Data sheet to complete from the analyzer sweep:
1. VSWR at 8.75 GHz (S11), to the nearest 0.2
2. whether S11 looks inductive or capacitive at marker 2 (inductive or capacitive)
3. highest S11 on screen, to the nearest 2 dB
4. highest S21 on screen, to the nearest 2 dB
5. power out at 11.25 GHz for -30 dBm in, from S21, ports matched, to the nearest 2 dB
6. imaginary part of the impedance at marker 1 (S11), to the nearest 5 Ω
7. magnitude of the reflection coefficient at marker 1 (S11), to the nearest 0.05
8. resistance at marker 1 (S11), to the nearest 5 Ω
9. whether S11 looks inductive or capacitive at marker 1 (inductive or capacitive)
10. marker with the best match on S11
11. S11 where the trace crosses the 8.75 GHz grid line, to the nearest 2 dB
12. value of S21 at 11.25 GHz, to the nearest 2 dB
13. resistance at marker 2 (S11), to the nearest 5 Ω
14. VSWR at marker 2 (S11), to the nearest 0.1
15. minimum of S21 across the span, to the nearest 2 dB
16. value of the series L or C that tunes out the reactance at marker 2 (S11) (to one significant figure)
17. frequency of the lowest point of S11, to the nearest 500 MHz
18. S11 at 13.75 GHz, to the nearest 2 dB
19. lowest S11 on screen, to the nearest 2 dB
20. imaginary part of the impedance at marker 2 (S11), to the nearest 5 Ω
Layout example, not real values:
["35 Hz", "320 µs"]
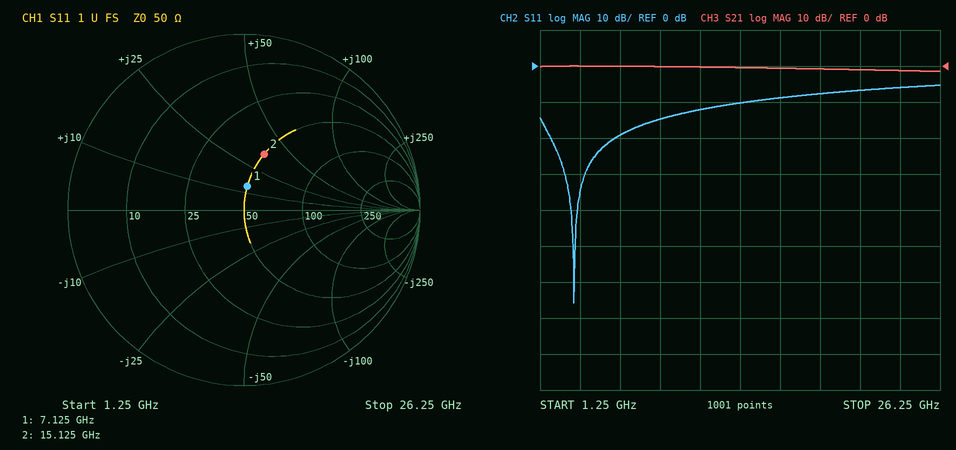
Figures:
["1.4", "inductive", "-6 dB", "0 dB", "-30 dBm", "+15 Ω", "0.15", "50 Ω", "inductive", "marker 1", "-14 dB", "0 dB", "50 Ω", "2.0", "-2 dB", "300 fF", "3.5 GHz", "-10 dB", "-66 dB", "+35 Ω"]
